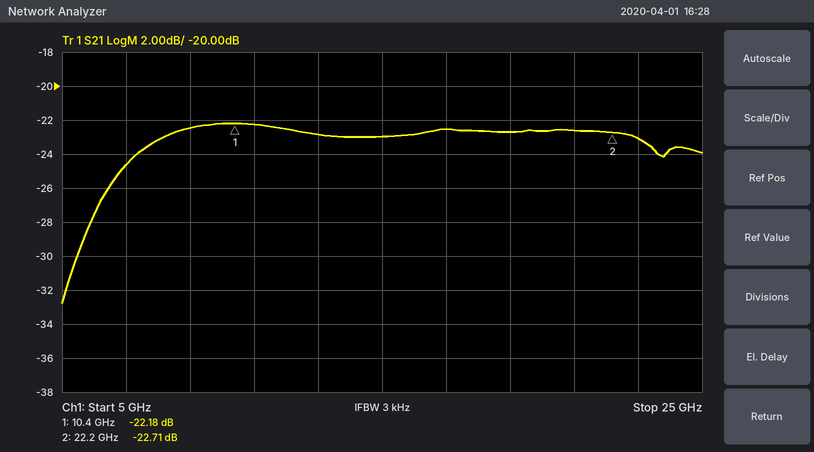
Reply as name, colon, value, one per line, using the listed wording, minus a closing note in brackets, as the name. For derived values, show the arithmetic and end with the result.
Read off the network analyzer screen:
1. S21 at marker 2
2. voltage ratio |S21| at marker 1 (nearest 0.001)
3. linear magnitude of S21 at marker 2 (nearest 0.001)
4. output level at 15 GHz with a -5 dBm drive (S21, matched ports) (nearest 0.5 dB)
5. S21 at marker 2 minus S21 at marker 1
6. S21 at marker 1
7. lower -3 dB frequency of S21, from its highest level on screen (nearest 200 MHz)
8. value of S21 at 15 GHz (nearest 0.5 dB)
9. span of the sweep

S21 at marker 2: -22.71 dB
voltage ratio |S21| at marker 1: 10^(-22.18/20) ≈ 0.078
linear magnitude of S21 at marker 2: 10^(-22.71/20) ≈ 0.073
output level at 15 GHz with a -5 dBm drive (S21, matched ports): -5 dBm + (-23.0 dB) = -28.0 dBm
S21 at marker 2 minus S21 at marker 1: -22.71 − (-22.18) = -0.53 dB
S21 at marker 1: -22.18 dB
lower -3 dB frequency of S21, from its highest level on screen: 6.8 GHz
value of S21 at 15 GHz: -23.0 dB
span of the sweep: 20 GHz
